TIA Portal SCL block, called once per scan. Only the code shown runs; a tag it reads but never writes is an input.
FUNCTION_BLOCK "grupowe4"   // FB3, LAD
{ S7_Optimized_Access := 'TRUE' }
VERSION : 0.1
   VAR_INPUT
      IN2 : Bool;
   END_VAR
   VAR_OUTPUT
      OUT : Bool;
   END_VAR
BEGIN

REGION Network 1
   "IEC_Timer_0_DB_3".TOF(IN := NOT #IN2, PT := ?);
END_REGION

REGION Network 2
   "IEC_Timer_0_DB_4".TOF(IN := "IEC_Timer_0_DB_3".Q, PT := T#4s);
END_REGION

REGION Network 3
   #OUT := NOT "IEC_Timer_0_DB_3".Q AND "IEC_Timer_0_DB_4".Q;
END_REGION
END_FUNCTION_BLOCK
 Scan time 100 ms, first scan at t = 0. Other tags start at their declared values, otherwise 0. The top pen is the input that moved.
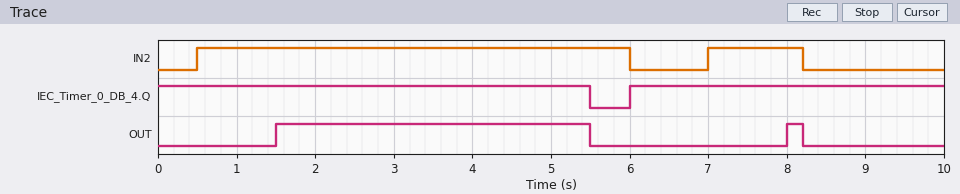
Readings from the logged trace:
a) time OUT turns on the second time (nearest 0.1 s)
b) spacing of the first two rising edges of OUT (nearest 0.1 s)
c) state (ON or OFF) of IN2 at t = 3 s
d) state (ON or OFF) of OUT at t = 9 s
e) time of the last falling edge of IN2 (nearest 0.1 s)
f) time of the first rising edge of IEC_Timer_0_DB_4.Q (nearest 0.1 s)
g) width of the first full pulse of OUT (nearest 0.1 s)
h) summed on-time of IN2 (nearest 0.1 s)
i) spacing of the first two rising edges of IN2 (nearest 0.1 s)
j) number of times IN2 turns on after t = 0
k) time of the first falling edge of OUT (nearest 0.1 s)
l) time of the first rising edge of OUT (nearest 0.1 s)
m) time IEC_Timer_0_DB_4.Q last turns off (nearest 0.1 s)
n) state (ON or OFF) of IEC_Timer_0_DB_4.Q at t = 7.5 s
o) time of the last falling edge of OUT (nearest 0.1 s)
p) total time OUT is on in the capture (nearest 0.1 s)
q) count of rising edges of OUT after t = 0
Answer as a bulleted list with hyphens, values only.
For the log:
- 8.0 s
- 6.5 s
- ON
- OFF
- 8.2 s
- 6.0 s
- 4.0 s
- 6.7 s
- 6.5 s
- 2
- 5.5 s
- 1.5 s
- 5.5 s
- ON
- 8.2 s
- 4.2 s
- 2
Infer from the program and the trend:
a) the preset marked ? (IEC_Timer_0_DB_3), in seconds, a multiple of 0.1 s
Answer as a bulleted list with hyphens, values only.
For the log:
- 1.0 s
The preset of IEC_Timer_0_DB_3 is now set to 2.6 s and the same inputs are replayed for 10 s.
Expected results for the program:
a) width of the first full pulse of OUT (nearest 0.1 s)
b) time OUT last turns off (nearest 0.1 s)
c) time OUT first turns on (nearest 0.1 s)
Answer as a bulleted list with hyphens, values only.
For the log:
- 2.9 s
- 6.0 s
- 3.1 s
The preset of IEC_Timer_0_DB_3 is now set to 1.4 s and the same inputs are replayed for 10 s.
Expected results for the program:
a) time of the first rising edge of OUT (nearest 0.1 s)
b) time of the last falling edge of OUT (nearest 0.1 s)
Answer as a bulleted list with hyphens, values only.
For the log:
- 1.9 s
- 5.9 s
